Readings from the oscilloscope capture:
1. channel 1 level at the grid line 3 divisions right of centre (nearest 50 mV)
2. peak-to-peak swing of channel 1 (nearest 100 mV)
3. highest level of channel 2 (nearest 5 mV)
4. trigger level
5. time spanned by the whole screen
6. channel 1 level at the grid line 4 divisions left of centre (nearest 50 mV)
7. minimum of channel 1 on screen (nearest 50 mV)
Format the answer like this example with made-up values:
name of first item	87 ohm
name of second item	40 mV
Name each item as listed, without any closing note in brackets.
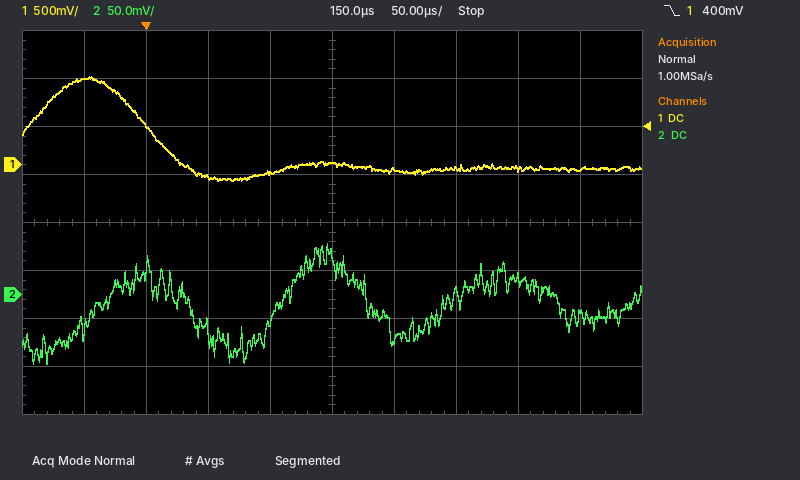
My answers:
channel 1 level at the grid line 3 divisions right of centre	-50 mV
peak-to-peak swing of channel 1	1.10 V
highest level of channel 2	55 mV
trigger level	400 mV
time spanned by the whole screen	500 µs
channel 1 level at the grid line 4 divisions left of centre	900 mV
minimum of channel 1 on screen	-150 mV
